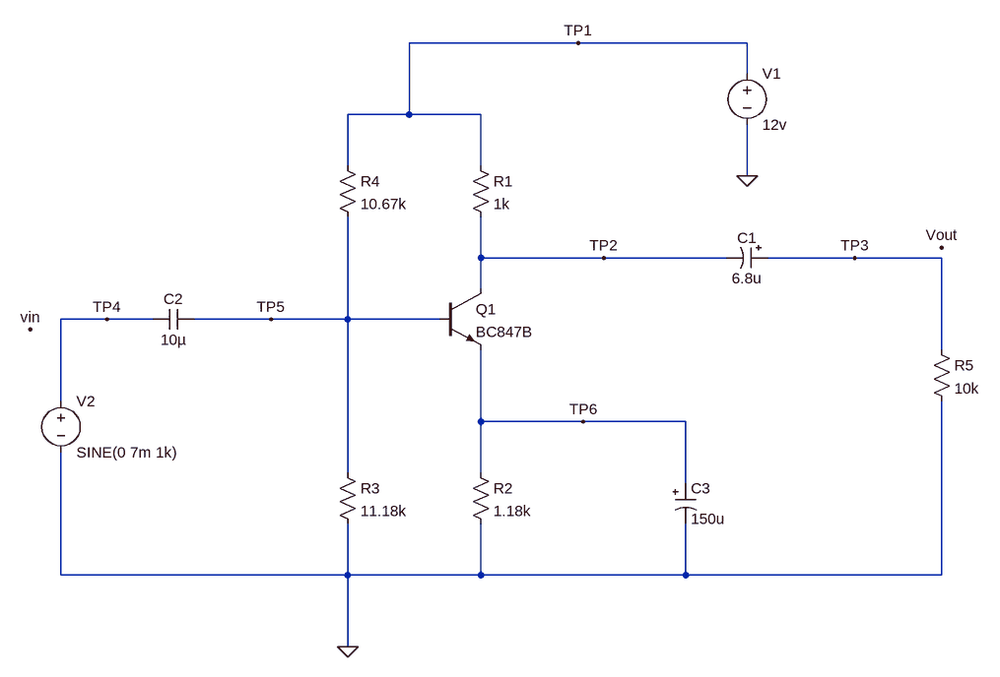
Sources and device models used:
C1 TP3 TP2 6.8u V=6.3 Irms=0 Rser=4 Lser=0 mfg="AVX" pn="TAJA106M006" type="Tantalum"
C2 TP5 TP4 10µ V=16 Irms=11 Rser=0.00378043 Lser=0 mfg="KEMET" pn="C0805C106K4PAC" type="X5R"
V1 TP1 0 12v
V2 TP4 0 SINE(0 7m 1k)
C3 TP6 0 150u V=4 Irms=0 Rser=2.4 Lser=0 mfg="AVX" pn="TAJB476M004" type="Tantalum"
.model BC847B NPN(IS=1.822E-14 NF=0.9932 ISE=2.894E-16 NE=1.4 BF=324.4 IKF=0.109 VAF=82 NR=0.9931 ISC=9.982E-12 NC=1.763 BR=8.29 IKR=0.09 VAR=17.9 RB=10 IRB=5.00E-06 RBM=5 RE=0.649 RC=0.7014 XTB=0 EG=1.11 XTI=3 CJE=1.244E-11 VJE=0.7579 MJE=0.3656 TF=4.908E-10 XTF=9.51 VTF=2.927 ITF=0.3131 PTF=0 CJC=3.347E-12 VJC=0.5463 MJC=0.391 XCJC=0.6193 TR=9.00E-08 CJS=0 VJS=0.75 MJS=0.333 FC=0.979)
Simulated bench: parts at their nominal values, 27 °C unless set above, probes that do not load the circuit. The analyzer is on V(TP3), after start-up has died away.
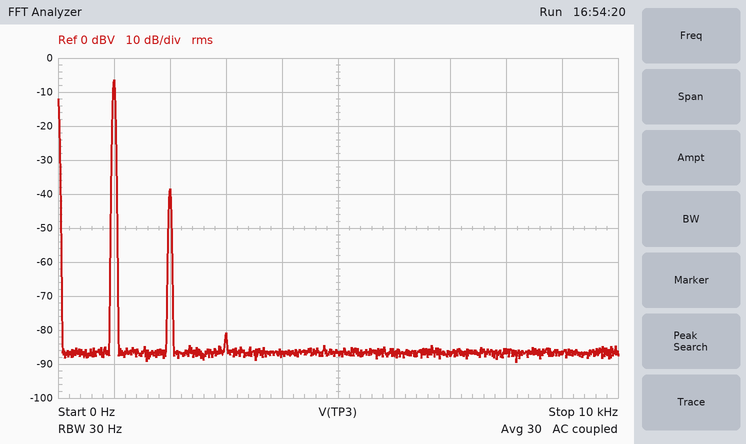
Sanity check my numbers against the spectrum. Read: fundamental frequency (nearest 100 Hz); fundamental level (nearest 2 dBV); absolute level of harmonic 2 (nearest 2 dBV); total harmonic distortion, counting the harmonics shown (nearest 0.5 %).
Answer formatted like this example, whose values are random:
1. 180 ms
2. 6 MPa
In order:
1. 1.0 kHz
2. -6 dBV
3. -38 dBV
4. 2.5 %
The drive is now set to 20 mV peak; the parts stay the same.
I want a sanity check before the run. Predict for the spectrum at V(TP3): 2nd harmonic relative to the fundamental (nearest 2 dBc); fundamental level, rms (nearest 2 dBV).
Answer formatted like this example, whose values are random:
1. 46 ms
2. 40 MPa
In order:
1. -24 dBc
2. 2 dBV
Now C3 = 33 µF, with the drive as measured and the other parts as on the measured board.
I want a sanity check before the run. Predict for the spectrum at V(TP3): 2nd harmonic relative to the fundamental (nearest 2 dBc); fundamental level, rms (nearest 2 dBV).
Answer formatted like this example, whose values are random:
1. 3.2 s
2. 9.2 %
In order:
1. -34 dBc
2. -8 dBV
